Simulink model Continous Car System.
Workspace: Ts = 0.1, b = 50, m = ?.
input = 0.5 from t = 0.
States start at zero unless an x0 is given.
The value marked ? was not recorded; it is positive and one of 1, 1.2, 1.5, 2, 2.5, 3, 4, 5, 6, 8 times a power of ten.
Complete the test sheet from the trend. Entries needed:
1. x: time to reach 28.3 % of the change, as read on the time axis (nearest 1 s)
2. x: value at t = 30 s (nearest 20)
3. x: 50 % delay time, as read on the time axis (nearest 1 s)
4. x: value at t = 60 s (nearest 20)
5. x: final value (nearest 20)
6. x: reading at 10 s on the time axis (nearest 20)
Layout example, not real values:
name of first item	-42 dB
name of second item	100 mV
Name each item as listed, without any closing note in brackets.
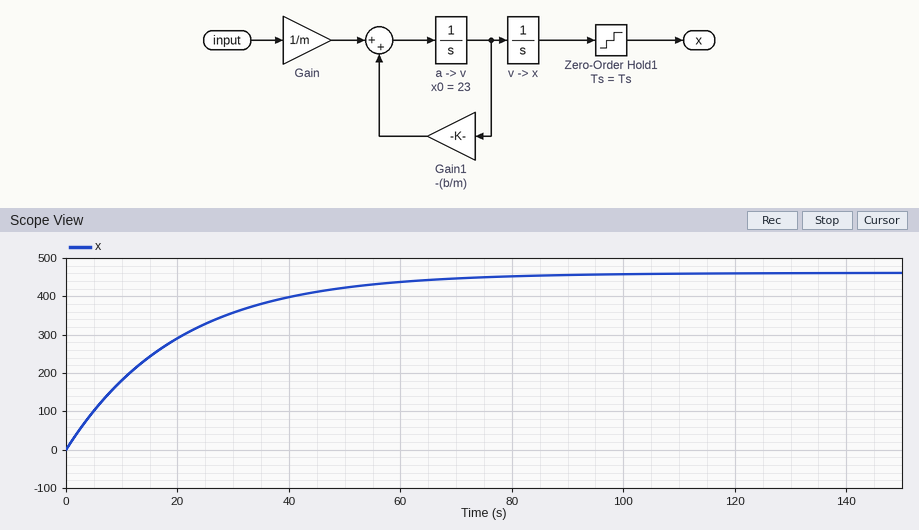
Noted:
x: time to reach 28.3 % of the change, as read on the time axis	7 s
x: value at t = 30 s	360
x: 50 % delay time, as read on the time axis	14 s
x: value at t = 60 s	440
x: final value	460
x: reading at 10 s on the time axis	180
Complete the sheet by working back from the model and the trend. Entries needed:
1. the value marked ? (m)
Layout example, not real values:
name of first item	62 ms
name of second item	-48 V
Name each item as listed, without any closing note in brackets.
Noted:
the value marked ?	1000
